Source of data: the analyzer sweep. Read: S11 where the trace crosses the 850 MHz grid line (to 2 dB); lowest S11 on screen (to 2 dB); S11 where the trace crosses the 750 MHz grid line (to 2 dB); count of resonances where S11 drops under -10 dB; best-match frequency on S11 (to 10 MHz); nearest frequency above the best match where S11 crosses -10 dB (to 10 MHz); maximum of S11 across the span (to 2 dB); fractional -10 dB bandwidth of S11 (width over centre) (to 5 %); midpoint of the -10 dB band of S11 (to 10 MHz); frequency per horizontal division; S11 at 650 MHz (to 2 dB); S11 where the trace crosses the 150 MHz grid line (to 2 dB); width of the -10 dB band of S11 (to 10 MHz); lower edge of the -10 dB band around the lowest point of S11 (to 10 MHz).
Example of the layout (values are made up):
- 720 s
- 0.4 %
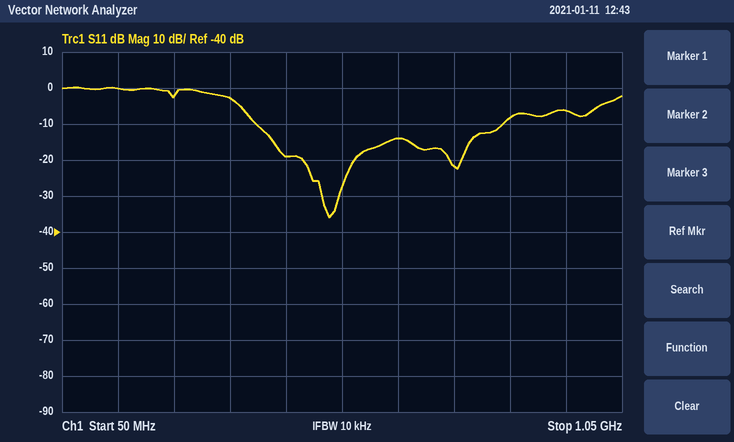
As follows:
- -8 dB
- -36 dB
- -22 dB
- 2
- 530 MHz
- 840 MHz
- 0 dB
- 70 %
- 620 MHz
- 100 MHz
- -14 dB
- 0 dB
- 440 MHz
- 400 MHz
